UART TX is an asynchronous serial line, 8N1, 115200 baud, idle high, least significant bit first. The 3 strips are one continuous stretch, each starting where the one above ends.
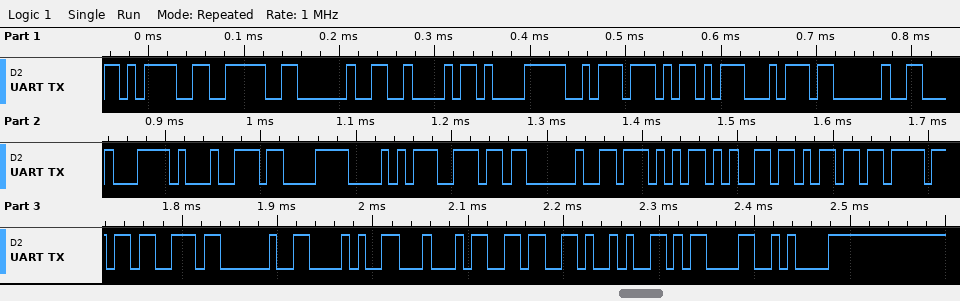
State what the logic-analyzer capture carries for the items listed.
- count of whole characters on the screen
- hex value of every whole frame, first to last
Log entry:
27
3D 3E 20 42 E1 BA AD 74 20 C4 91 C3 A8 6E 20 57 65 6D 6F 73 20 28 44 36 29 0D 0A
